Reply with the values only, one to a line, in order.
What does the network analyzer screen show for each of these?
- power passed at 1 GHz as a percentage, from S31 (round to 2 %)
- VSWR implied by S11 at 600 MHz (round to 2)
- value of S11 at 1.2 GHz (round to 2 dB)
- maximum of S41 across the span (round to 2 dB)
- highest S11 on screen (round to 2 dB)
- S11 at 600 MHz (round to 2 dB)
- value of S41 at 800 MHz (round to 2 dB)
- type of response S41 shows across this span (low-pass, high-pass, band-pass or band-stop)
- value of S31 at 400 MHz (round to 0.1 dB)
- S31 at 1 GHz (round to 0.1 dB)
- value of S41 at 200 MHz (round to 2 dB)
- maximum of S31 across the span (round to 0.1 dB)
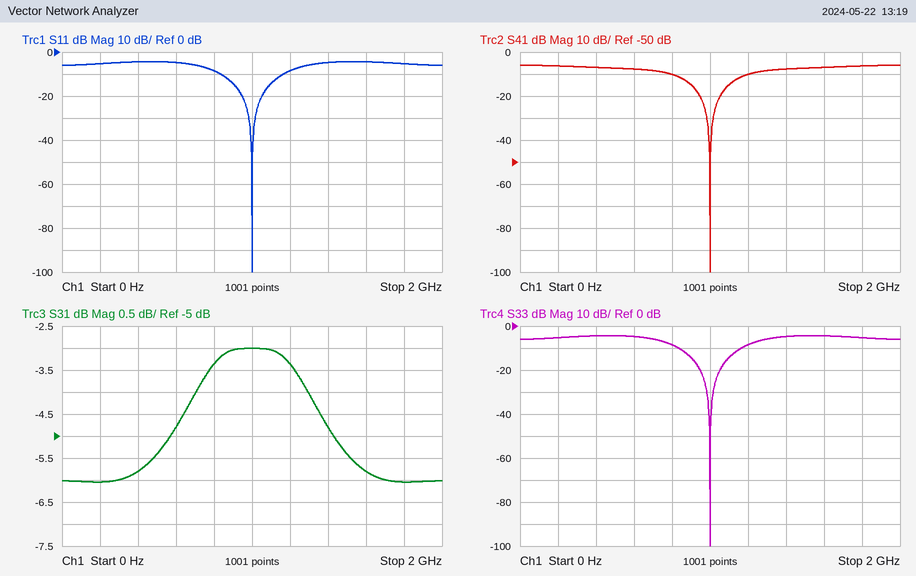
50 %
4
-8 dB
-6 dB
-4 dB
-4 dB
-10 dB
band-stop
-5.8 dB
-3.0 dB
-6 dB
-3.0 dB
